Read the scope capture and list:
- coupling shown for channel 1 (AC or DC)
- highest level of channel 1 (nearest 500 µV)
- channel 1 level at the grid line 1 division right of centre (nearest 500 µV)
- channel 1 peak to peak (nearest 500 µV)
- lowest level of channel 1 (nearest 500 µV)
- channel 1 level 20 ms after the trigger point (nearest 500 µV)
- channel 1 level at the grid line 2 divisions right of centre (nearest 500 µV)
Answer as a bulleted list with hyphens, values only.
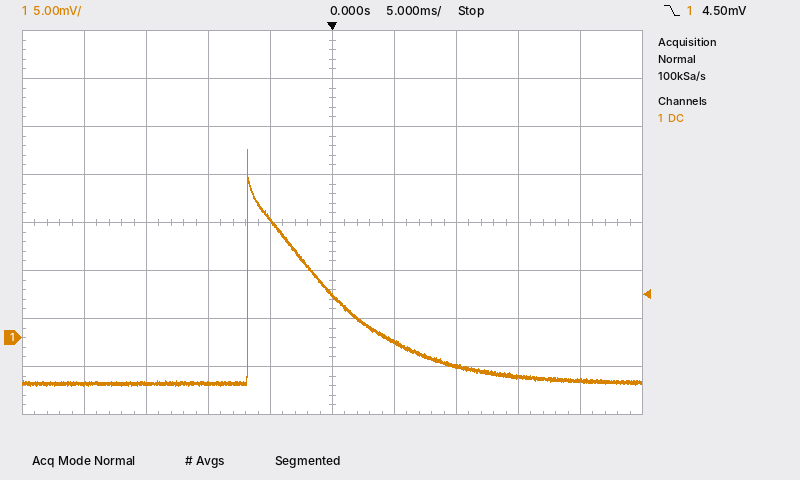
- DC
- 19.5 mV
- -500 µV
- 24.5 mV
- -5.0 mV
- -4.5 mV
- -3.0 mV
